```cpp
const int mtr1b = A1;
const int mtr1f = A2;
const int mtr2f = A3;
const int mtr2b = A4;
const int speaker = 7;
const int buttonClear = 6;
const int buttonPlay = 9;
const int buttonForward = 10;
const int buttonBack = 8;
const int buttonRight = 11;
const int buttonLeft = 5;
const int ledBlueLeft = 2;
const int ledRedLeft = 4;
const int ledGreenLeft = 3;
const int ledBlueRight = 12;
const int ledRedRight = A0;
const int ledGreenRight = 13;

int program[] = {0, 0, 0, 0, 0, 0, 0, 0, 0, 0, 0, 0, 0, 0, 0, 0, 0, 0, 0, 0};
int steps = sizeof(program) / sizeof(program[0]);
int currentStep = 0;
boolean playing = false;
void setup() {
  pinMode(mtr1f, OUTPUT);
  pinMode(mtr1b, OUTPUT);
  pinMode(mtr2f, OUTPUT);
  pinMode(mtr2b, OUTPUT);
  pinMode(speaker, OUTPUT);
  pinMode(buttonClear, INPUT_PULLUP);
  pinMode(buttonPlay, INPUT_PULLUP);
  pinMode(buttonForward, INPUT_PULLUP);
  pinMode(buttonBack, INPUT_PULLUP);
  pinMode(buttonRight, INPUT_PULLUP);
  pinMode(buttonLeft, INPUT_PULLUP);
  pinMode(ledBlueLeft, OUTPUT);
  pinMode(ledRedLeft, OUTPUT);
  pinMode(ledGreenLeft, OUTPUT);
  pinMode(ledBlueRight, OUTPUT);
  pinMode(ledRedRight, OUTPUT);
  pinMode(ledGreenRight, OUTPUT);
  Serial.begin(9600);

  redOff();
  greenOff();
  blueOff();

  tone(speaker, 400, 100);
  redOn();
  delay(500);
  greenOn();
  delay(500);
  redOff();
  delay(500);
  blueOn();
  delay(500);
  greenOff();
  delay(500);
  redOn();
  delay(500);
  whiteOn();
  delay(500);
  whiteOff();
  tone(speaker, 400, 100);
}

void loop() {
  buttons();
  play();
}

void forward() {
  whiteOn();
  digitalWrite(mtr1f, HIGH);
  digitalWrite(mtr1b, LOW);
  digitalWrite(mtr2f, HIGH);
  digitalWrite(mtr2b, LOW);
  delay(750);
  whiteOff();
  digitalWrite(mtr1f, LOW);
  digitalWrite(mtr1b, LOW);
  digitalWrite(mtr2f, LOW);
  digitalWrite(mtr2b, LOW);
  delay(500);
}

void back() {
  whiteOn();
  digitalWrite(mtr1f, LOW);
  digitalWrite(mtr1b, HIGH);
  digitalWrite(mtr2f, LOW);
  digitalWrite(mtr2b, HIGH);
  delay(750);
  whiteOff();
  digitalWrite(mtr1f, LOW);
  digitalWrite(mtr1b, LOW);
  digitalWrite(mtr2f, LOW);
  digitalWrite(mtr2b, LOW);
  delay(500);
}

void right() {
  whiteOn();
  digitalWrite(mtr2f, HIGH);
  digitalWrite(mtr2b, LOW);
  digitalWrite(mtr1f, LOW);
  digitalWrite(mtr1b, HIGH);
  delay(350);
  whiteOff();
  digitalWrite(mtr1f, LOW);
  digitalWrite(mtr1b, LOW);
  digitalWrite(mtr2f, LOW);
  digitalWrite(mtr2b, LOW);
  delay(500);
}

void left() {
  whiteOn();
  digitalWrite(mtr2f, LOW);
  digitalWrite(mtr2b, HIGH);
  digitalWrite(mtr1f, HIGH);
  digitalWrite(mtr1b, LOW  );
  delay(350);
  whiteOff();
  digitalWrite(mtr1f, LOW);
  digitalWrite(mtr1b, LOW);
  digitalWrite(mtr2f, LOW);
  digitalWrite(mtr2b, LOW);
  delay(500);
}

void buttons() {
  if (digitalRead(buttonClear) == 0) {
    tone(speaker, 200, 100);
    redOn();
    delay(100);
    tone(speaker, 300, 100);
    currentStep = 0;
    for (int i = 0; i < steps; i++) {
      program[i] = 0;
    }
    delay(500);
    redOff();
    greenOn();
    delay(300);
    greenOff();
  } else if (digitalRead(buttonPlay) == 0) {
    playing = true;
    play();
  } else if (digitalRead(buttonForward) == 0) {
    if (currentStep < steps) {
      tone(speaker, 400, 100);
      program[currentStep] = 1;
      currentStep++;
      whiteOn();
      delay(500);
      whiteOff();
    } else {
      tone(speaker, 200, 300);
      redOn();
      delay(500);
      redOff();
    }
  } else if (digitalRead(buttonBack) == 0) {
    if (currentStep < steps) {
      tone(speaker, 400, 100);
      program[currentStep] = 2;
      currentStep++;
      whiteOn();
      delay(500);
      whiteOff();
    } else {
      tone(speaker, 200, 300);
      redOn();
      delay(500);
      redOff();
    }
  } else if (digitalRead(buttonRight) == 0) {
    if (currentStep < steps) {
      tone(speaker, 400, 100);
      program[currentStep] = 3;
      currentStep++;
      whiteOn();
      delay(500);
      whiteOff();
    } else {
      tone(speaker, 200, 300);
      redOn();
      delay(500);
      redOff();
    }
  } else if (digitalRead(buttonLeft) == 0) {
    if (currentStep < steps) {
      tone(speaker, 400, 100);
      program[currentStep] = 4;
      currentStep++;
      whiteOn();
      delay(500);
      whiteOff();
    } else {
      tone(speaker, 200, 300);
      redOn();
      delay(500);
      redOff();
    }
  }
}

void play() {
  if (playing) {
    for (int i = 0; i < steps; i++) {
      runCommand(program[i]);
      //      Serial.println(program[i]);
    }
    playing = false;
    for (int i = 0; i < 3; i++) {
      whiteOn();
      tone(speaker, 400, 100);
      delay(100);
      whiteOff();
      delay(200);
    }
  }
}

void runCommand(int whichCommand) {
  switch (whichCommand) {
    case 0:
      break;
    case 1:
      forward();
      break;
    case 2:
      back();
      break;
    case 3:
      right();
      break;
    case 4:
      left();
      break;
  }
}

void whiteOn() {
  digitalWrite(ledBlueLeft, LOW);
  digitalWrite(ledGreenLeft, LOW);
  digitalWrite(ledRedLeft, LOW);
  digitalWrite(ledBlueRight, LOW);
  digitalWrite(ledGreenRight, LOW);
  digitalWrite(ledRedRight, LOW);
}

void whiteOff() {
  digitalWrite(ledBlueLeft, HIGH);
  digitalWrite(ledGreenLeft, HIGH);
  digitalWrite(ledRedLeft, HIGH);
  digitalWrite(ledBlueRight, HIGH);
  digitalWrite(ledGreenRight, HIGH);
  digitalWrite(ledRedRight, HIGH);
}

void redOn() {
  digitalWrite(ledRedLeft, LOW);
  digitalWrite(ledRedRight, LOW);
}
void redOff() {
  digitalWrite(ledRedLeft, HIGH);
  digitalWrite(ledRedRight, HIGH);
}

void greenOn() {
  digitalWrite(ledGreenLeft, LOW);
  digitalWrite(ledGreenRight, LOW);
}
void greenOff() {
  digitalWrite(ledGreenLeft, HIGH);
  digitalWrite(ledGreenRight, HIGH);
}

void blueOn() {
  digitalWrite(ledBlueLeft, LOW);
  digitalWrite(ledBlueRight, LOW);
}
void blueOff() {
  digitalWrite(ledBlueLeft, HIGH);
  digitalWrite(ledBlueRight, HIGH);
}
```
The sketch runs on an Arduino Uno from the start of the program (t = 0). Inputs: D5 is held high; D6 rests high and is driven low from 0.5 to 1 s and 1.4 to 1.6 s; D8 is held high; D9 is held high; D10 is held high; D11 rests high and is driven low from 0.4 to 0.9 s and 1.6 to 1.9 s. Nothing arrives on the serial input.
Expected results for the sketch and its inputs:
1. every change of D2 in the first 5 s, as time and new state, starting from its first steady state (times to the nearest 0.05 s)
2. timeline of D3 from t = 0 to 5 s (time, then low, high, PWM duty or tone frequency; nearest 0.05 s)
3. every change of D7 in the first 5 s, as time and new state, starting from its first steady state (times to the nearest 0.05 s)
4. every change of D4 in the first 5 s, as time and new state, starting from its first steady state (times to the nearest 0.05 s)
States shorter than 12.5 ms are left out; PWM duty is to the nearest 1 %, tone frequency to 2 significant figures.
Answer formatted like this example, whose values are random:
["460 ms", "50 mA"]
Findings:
["0 s high; 1.5 s low; 3.5 s high", "0 s high; 0.5 s low; 2 s high; 3 s low; 3.5 s high", "0 s tone 400 Hz; 0.1 s low; 3.5 s tone 400 Hz; 3.6 s low", "0 s low; 1 s high; 2.5 s low; 3.5 s high"]
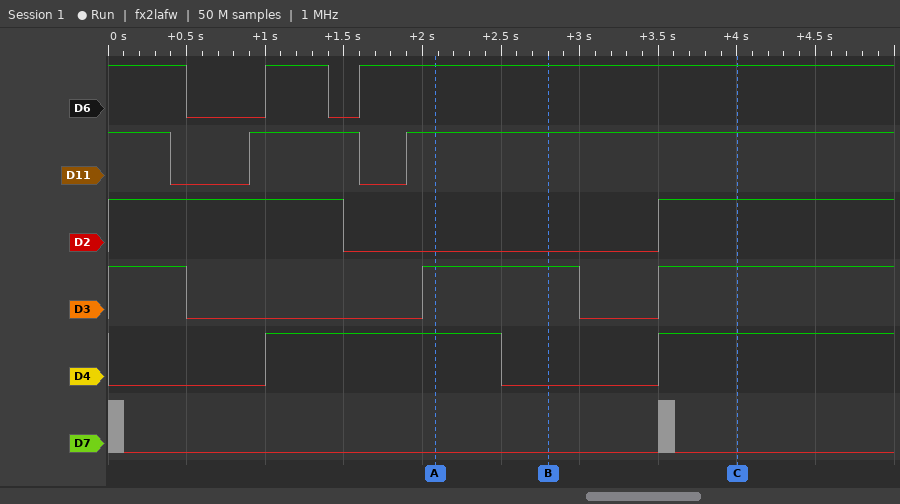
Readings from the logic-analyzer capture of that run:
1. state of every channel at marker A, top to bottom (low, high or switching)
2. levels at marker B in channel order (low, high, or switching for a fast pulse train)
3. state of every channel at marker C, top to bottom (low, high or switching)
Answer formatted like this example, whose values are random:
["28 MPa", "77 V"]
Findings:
["D6 high, D11 high, D2 low, D3 high, D4 high, D7 low", "D6 high, D11 high, D2 low, D3 high, D4 low, D7 low", "D6 high, D11 high, D2 high, D3 high, D4 high, D7 low"]
